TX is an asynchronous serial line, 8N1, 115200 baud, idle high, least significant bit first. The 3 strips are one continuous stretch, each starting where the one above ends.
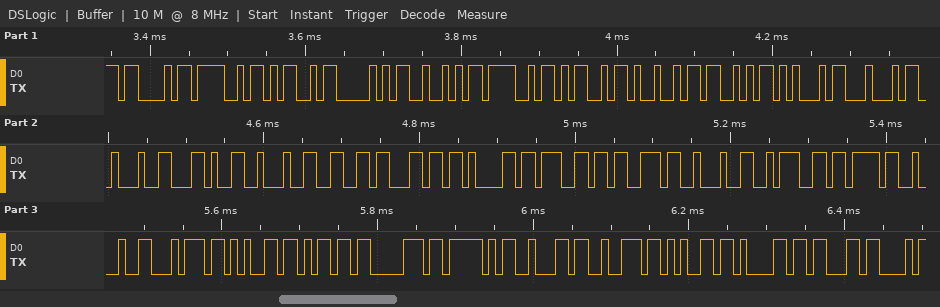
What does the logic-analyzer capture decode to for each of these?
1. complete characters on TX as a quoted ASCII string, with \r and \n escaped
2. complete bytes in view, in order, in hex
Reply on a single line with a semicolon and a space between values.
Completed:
"COMPROMISED\",\"flags\":{\"temp_breac"; 43 4F 4D 50 52 4F 4D 49 53 45 44 22 2C 22 66 6C 61 67 73 22 3A 7B 22 74 65 6D 70 5F 62 72 65 61 63
